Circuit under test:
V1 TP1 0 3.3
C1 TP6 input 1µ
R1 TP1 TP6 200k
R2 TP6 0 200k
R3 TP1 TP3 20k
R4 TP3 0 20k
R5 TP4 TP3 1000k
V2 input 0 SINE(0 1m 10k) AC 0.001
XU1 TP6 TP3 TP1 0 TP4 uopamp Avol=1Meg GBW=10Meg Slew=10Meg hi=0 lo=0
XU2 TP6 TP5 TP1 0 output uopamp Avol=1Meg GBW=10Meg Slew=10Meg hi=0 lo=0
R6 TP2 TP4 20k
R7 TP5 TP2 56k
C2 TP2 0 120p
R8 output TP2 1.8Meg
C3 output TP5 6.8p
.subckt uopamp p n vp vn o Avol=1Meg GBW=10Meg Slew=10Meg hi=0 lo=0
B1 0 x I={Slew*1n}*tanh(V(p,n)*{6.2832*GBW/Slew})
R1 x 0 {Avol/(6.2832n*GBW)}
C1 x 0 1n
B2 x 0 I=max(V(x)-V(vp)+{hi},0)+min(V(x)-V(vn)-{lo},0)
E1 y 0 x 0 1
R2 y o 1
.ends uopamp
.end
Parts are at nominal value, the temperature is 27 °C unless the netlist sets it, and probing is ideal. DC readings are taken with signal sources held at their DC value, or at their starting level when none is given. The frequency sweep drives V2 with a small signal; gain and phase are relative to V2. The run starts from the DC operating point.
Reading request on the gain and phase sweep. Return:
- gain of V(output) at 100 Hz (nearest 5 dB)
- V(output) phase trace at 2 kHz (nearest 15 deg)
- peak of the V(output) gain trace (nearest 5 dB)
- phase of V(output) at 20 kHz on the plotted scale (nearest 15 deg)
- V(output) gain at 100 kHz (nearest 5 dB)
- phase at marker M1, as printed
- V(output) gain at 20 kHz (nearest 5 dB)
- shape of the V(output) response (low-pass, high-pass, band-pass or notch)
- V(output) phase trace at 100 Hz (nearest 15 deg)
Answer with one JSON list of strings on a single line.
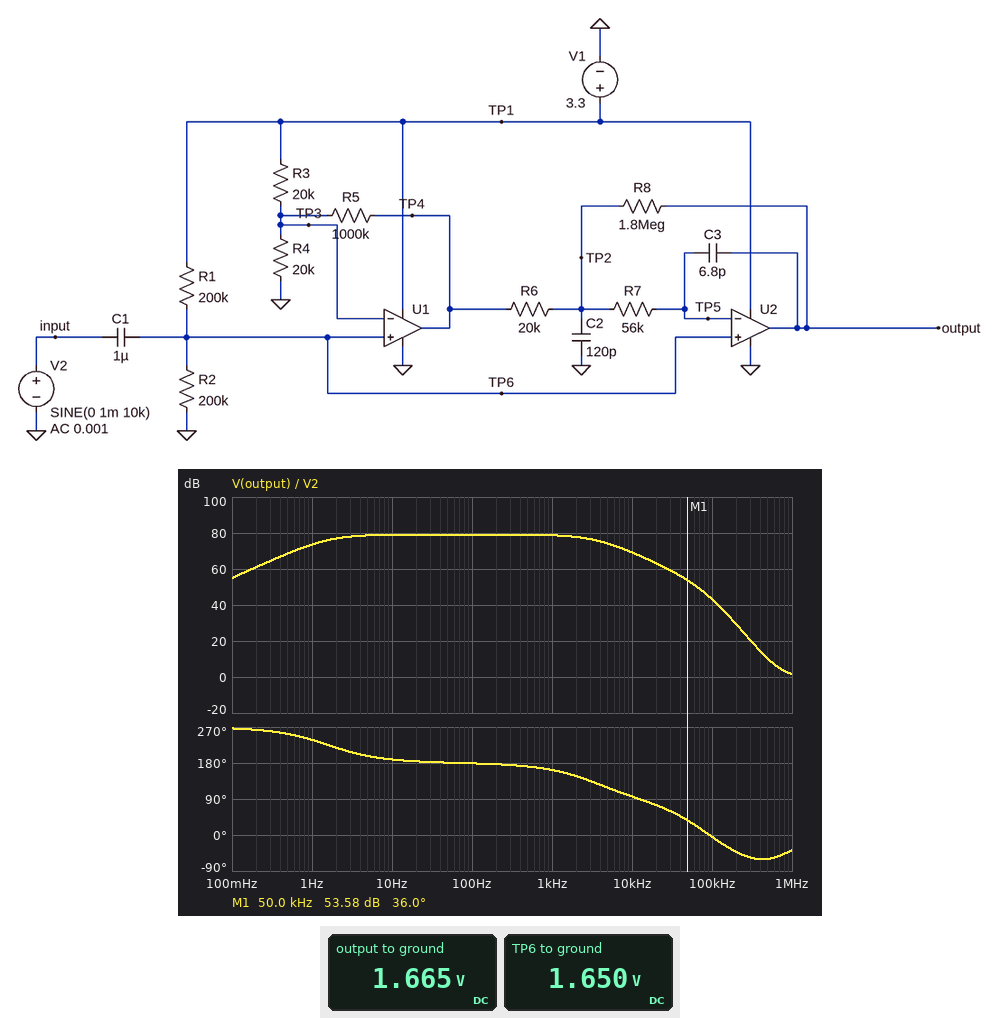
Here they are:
["80 dB", "150 deg", "80 dB", "75 deg", "45 dB", "36.0 deg", "65 dB", "band-pass", "180 deg"]
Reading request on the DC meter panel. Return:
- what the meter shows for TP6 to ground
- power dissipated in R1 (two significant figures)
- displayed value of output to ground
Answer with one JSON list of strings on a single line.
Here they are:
["1.650 V", "14 µW", "1.665 V"]
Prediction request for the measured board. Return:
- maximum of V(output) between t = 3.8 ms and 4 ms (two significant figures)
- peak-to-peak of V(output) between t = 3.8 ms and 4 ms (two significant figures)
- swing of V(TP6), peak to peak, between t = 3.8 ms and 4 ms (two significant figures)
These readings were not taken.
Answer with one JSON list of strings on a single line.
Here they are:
["3.3 V", "3.3 V", "2.0 mV"]
